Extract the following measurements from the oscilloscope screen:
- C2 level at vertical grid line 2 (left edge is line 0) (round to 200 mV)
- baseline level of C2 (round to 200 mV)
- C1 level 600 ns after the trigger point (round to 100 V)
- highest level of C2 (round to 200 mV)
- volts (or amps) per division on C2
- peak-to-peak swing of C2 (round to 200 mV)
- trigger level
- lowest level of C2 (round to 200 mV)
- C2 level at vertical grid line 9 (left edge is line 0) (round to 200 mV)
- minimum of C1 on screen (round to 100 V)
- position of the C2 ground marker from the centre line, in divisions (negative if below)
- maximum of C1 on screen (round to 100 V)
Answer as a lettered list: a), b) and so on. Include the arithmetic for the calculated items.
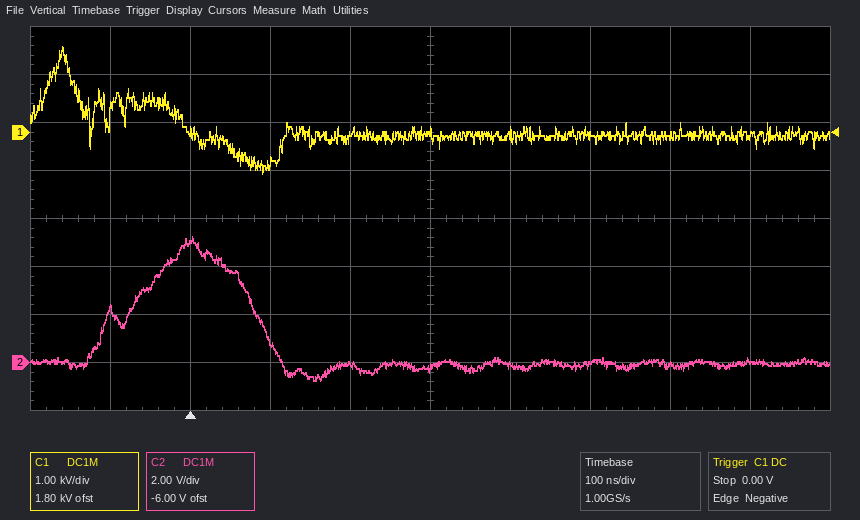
a) 5.0 V
b) 0.0 V
c) -100 V
d) 5.2 V
e) 2 V
f) 5.2 V − (-800 mV) = 6.0 V
g) 0.00 V
h) -800 mV
i) 0.0 V
j) -900 V
k) -3.0 div
l) 1.8 kV
